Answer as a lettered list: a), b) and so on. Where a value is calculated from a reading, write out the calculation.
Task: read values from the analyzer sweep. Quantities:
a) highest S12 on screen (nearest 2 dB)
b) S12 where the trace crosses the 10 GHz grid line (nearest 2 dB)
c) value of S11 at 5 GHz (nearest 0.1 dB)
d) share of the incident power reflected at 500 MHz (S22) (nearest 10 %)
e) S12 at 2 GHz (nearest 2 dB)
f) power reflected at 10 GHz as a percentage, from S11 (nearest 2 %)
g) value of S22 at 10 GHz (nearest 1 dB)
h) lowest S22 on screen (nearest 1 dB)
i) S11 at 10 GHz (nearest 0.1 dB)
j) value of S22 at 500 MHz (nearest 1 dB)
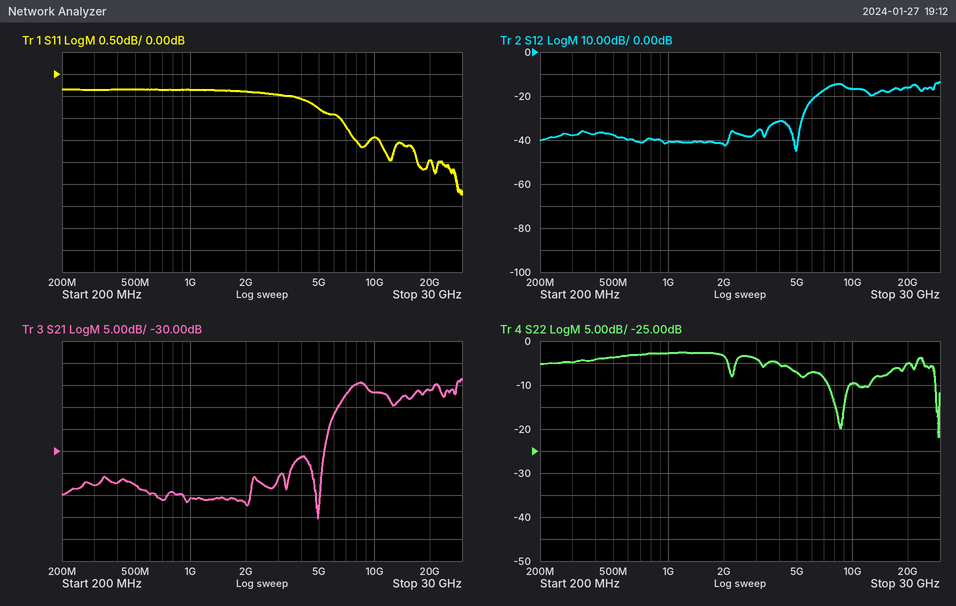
a) -14 dB
b) -16 dB
c) -0.8 dB
d) 10^(-4/10) ≈ 40 %
e) -42 dB
f) 10^(-1.4/10) ≈ 72 %
g) -10 dB
h) -22 dB
i) -1.4 dB
j) -4 dB
